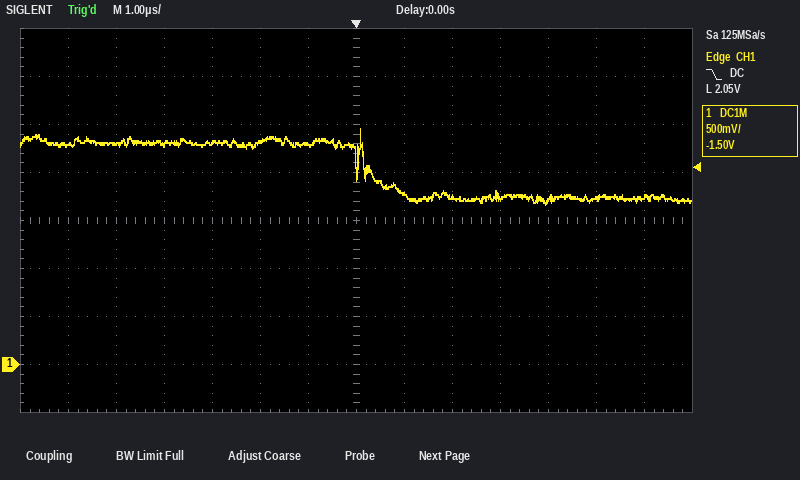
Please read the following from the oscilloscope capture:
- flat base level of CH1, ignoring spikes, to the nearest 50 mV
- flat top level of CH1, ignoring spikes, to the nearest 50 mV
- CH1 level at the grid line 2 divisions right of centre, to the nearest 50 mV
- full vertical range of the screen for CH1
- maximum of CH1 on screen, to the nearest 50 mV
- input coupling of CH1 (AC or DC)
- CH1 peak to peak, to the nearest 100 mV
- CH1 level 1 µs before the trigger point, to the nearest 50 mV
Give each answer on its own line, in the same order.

1.75 V
2.30 V
1.75 V
4 V
2.45 V
DC
800 mV
2.30 V
